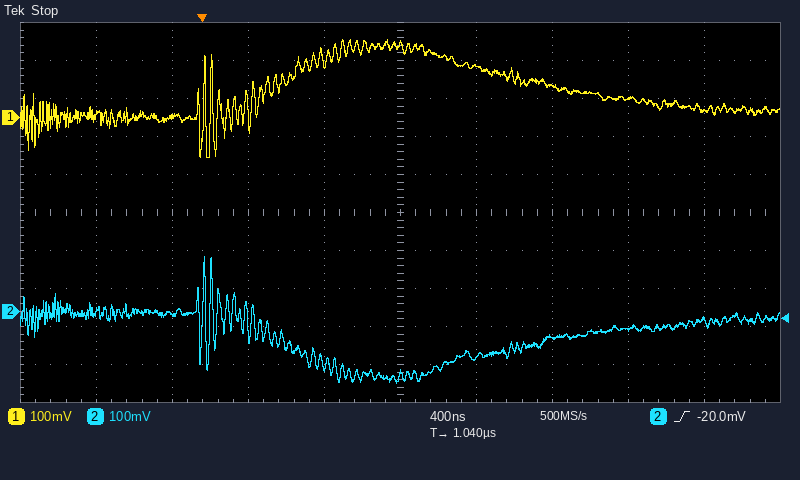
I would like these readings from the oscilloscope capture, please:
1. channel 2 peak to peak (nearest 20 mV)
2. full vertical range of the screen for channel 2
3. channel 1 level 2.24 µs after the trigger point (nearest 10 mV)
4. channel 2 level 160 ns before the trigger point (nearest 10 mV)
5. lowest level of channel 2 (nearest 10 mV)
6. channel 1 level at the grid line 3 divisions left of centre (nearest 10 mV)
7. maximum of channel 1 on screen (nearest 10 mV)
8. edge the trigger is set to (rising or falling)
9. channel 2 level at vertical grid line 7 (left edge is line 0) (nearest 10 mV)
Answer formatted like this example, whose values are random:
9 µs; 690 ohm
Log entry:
340 mV; 1 V; 50 mV; -10 mV; -190 mV; 0 mV; 210 mV; rising; -70 mV
